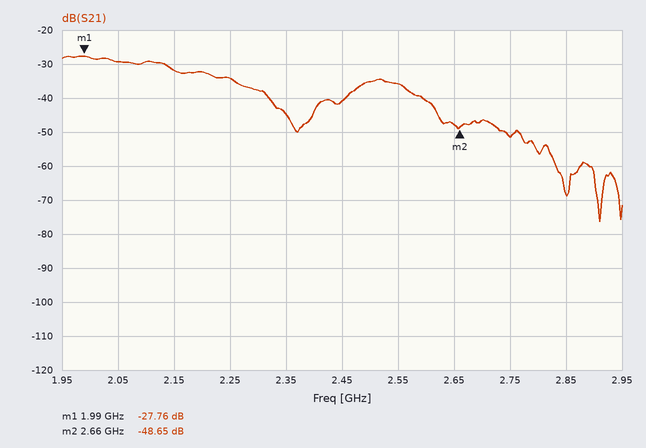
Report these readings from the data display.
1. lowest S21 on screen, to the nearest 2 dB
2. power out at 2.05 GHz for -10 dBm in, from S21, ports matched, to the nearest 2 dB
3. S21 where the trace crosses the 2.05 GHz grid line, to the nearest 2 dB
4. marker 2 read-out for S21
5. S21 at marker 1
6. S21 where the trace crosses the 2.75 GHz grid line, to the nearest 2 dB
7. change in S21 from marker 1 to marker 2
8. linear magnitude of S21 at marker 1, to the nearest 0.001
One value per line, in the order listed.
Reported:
-76 dB
-40 dBm
-30 dB
-48.65 dB
-27.76 dB
-52 dB
-20.89 dB
0.041
